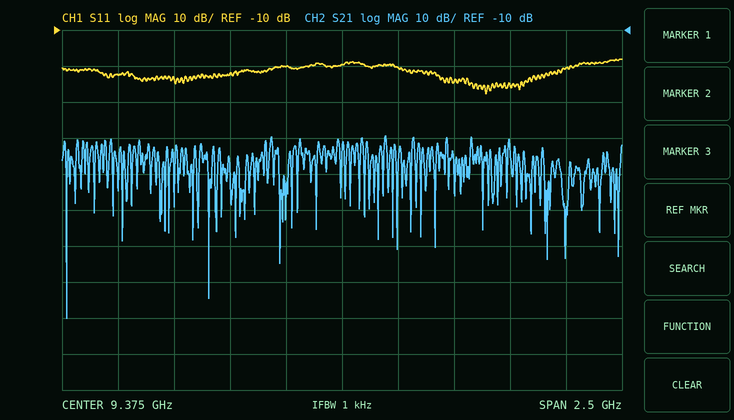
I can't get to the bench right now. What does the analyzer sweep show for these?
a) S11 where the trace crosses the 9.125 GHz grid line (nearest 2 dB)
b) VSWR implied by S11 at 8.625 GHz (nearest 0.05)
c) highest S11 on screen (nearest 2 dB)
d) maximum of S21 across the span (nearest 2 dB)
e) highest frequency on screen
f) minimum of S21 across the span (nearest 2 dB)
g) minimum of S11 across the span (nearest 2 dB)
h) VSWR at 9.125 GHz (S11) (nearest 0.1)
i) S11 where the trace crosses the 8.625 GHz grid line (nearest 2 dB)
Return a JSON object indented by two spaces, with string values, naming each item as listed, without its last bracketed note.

{
  "S11 where the trace crosses the 9.125 GHz grid line": "-20 dB",
  "VSWR implied by S11 at 8.625 GHz": "1.15",
  "highest S11 on screen": "-18 dB",
  "maximum of S21 across the span": "-40 dB",
  "highest frequency on screen": "10.625 GHz",
  "minimum of S21 across the span": "-90 dB",
  "minimum of S11 across the span": "-28 dB",
  "VSWR at 9.125 GHz (S11)": "1.2",
  "S11 where the trace crosses the 8.625 GHz grid line": "-24 dB"
}
